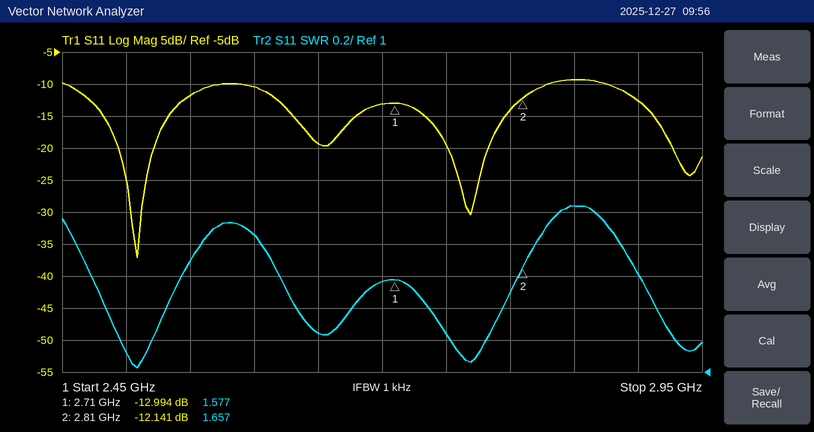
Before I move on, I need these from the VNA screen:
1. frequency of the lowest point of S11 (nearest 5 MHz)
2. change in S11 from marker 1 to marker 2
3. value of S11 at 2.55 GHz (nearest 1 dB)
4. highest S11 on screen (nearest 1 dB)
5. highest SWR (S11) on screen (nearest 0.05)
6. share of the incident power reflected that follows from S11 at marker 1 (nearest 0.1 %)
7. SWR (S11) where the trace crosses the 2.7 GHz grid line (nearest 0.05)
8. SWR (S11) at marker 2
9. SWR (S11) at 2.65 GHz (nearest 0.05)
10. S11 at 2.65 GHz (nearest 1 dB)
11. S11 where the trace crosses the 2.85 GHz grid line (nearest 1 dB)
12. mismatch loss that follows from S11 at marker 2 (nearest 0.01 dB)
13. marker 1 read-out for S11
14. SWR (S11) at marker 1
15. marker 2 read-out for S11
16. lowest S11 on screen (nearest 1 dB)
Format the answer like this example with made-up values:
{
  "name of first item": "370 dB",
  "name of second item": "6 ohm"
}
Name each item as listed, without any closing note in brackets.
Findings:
{
  "frequency of the lowest point of S11": "2.510 GHz",
  "change in S11 from marker 1 to marker 2": "0.853 dB",
  "value of S11 at 2.55 GHz": "-12 dB",
  "highest S11 on screen": "-9 dB",
  "highest SWR (S11) on screen": "2.05",
  "share of the incident power reflected that follows from S11 at marker 1": "5.0 %",
  "SWR (S11) where the trace crosses the 2.7 GHz grid line": "1.55",
  "SWR (S11) at marker 2": "1.657",
  "SWR (S11) at 2.65 GHz": "1.25",
  "S11 at 2.65 GHz": "-19 dB",
  "S11 where the trace crosses the 2.85 GHz grid line": "-9 dB",
  "mismatch loss that follows from S11 at marker 2": "0.27 dB",
  "marker 1 read-out for S11": "-12.994 dB",
  "SWR (S11) at marker 1": "1.577",
  "marker 2 read-out for S11": "-12.141 dB",
  "lowest S11 on screen": "-37 dB"
}
